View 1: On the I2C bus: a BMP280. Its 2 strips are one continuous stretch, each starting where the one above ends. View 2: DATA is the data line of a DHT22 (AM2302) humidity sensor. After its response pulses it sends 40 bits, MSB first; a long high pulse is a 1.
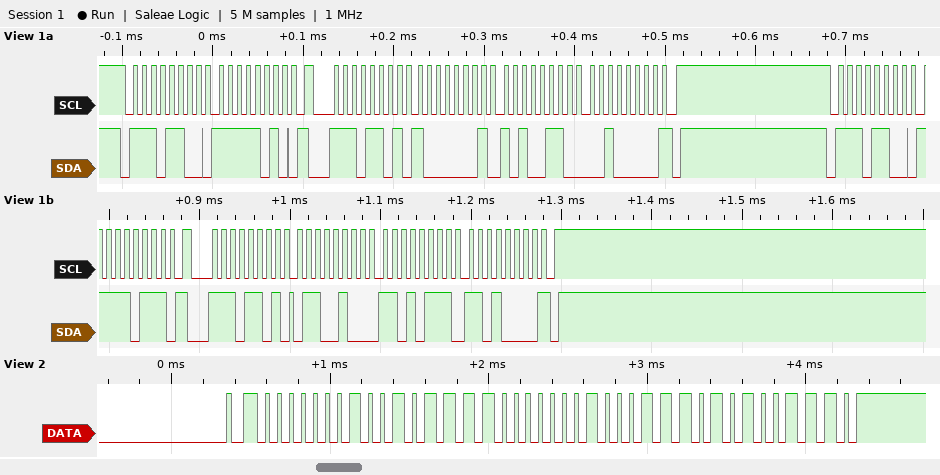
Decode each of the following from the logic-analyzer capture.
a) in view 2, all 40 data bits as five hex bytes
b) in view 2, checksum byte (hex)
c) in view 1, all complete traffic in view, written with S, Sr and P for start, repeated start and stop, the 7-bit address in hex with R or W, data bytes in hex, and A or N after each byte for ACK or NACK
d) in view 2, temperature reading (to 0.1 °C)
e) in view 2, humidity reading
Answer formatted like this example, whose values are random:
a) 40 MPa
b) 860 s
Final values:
a) 01 2F 01 1D 4E
b) 0x4E
c) S 76W A FA A Sr 76R A 81 A A6 A 20 N P S 76W A F7 A Sr 76R A 64 A D7 A D0 N P
d) 28.5 °C
e) 30.3 %
